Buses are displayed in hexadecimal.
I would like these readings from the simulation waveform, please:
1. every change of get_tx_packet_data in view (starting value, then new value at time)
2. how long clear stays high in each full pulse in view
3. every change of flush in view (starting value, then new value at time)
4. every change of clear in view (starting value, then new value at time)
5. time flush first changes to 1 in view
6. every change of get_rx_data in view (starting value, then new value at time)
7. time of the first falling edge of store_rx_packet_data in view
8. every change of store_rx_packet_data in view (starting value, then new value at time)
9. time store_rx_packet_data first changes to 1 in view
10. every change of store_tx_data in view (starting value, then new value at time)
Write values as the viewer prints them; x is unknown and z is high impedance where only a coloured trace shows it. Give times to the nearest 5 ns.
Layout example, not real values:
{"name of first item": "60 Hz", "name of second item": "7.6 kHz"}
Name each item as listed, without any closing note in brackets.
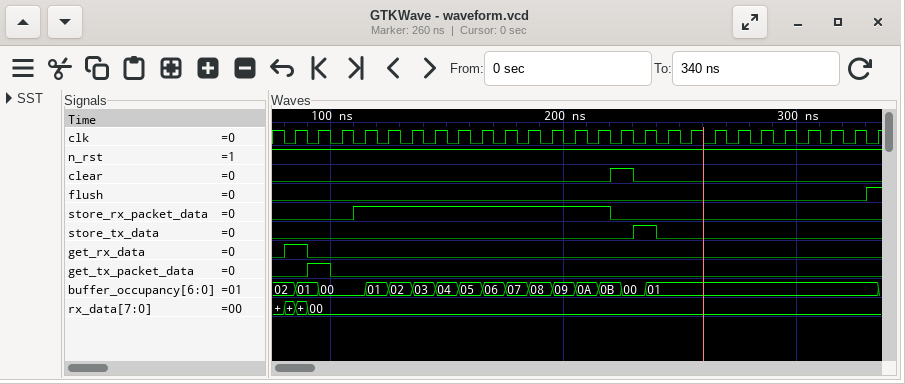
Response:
{"every change of get_tx_packet_data in view": "0, 1 at 90 ns, 0 at 100 ns", "how long clear stays high in each full pulse in view": "10 ns", "every change of flush in view": "0, 1 at 330 ns", "every change of clear in view": "0, 1 at 220 ns, 0 at 230 ns", "time flush first changes to 1 in view": "330 ns", "every change of get_rx_data in view": "0, 1 at 80 ns, 0 at 90 ns", "time of the first falling edge of store_rx_packet_data in view": "220 ns", "every change of store_rx_packet_data in view": "0, 1 at 110 ns, 0 at 220 ns", "time store_rx_packet_data first changes to 1 in view": "110 ns", "every change of store_tx_data in view": "0, 1 at 230 ns, 0 at 240 ns"}
